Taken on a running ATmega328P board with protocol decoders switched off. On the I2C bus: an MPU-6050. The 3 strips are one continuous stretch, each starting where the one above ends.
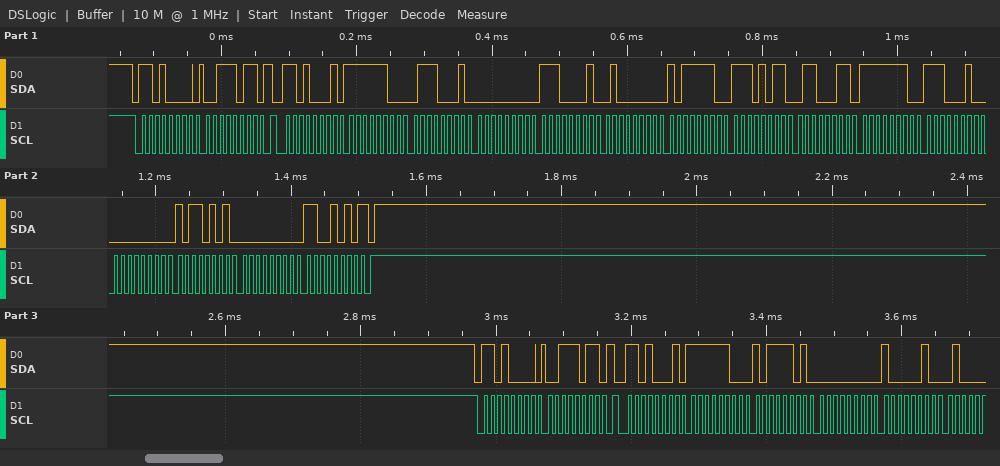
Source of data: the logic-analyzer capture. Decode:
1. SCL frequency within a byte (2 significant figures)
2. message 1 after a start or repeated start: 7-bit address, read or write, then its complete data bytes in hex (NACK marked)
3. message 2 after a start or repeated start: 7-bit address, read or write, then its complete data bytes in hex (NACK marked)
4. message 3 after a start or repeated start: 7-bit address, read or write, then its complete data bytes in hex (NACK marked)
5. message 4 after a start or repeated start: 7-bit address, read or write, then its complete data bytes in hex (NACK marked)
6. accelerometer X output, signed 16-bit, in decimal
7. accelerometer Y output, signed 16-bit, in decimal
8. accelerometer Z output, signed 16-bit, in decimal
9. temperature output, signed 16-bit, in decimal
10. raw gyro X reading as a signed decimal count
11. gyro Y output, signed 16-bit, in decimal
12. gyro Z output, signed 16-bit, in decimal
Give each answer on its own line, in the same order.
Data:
100 kHz
0x68 write: 3B
0x68 read: FC 71 00 E1 40 BE EB 63 FE E2 00 B5 00 CA NACK
0x68 write: 3B
0x68 read: FC BD 00 82
-911
225
16574
-5277
-286
181
202
